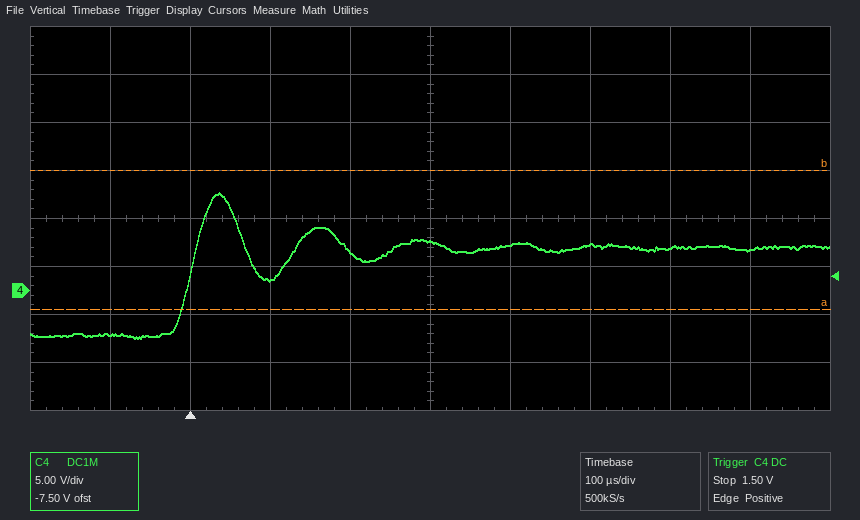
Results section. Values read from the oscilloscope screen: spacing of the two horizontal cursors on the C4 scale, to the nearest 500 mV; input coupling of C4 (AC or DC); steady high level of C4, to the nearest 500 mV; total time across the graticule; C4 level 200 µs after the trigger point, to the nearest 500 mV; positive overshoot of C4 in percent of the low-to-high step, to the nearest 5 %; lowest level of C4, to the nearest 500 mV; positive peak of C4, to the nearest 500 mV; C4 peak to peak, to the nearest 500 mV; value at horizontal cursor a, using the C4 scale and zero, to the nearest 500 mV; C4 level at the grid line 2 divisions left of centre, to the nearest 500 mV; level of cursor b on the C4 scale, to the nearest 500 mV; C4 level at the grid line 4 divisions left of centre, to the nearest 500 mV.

14.5 V
DC
4.5 V
1 ms
4.0 V
60 %
-5.0 V
10.0 V
15.0 V
-2.0 V
1.0 V
12.5 V
-4.5 V
